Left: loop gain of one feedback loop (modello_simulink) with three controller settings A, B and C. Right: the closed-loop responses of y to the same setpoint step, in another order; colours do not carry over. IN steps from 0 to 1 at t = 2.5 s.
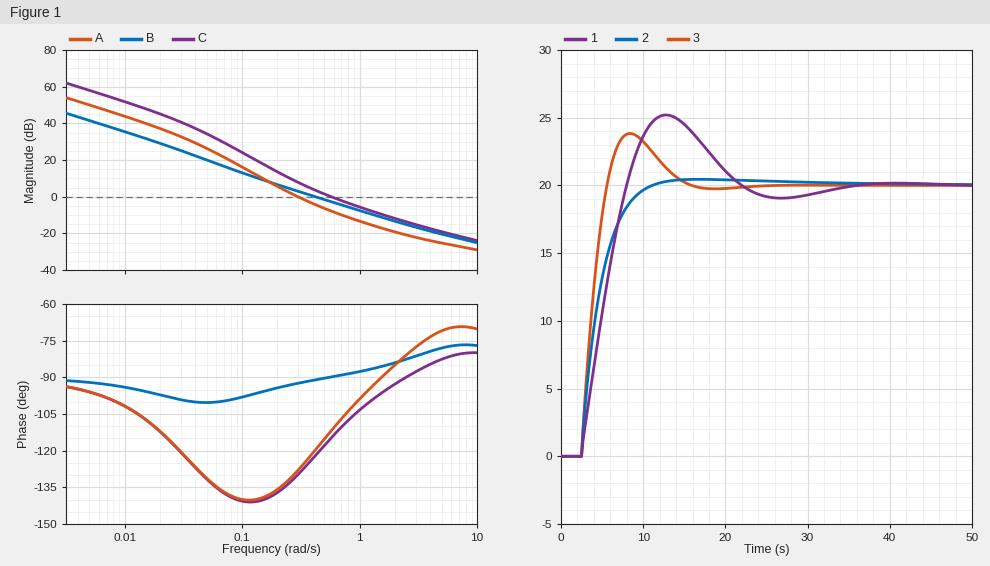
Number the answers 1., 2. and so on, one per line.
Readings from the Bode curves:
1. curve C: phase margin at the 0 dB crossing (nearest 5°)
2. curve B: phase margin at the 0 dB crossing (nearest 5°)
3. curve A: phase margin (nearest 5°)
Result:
1. 65°
2. 90°
3. 50°
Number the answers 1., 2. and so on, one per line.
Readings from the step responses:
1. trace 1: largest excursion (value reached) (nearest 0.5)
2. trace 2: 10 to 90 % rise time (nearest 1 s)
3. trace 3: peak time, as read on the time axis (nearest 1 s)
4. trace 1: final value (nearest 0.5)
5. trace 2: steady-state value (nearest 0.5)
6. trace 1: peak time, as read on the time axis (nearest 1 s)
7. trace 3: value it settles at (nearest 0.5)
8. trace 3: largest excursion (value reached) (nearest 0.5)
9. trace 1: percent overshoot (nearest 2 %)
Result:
1. 25.0
2. 5 s
3. 8 s
4. 20.0
5. 20.0
6. 13 s
7. 20.0
8. 24.0
9. 26 %
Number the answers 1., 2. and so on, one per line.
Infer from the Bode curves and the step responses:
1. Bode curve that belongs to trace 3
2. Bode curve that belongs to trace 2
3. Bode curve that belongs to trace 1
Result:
1. C
2. B
3. A
